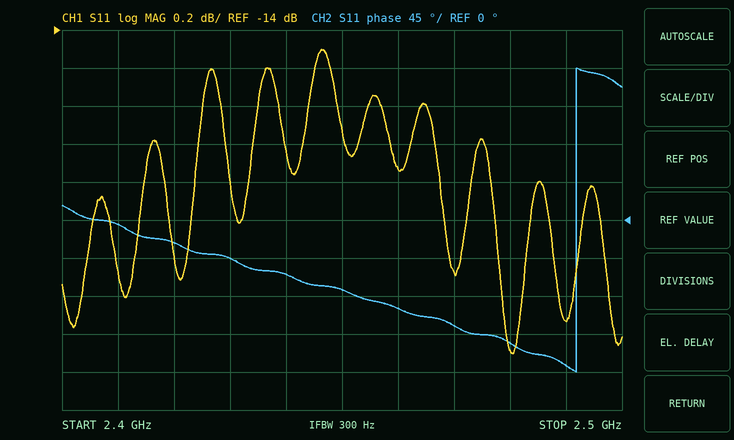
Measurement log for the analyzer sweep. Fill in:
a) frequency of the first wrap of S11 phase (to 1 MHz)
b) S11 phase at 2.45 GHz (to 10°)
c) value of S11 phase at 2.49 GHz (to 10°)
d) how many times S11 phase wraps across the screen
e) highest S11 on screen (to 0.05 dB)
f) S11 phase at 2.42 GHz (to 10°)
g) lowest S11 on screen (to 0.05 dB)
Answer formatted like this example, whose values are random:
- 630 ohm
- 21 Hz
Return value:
- 2.492 GHz
- -80°
- -170°
- 1
- -14.10 dB
- -30°
- -15.70 dB
